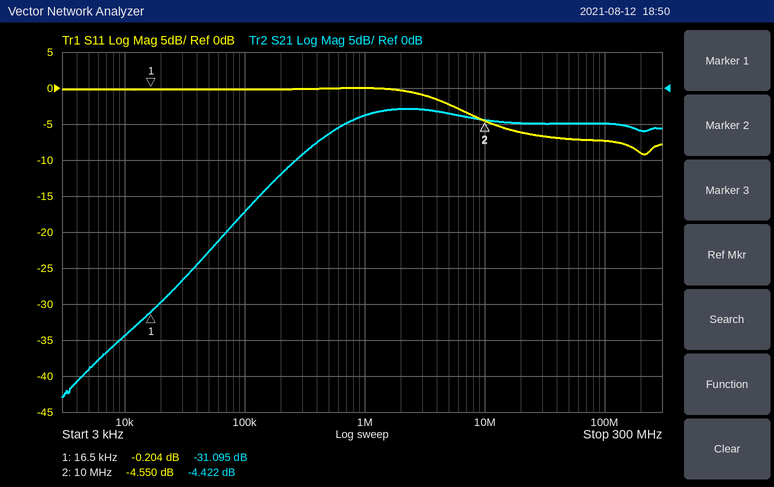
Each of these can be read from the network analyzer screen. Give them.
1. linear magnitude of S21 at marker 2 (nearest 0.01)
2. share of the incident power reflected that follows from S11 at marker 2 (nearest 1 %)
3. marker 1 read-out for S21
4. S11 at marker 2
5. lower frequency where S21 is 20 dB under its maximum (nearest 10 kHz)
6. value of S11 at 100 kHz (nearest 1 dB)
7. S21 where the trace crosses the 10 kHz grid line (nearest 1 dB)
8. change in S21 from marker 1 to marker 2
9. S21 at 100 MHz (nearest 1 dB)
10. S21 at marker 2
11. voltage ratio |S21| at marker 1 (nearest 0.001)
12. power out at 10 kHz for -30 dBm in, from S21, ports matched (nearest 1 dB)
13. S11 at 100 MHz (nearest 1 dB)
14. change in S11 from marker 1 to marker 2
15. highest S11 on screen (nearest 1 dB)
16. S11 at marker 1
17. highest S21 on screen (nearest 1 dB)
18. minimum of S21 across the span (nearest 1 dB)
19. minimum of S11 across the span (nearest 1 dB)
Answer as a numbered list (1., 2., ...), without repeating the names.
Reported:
1. 0.60
2. 35 %
3. -31.095 dB
4. -4.550 dB
5. 50 kHz
6. 0 dB
7. -34 dB
8. 26.673 dB
9. -5 dB
10. -4.422 dB
11. 0.028
12. -64 dBm
13. -7 dB
14. -4.346 dB
15. 0 dB
16. -0.204 dB
17. -3 dB
18. -43 dB
19. -9 dB
